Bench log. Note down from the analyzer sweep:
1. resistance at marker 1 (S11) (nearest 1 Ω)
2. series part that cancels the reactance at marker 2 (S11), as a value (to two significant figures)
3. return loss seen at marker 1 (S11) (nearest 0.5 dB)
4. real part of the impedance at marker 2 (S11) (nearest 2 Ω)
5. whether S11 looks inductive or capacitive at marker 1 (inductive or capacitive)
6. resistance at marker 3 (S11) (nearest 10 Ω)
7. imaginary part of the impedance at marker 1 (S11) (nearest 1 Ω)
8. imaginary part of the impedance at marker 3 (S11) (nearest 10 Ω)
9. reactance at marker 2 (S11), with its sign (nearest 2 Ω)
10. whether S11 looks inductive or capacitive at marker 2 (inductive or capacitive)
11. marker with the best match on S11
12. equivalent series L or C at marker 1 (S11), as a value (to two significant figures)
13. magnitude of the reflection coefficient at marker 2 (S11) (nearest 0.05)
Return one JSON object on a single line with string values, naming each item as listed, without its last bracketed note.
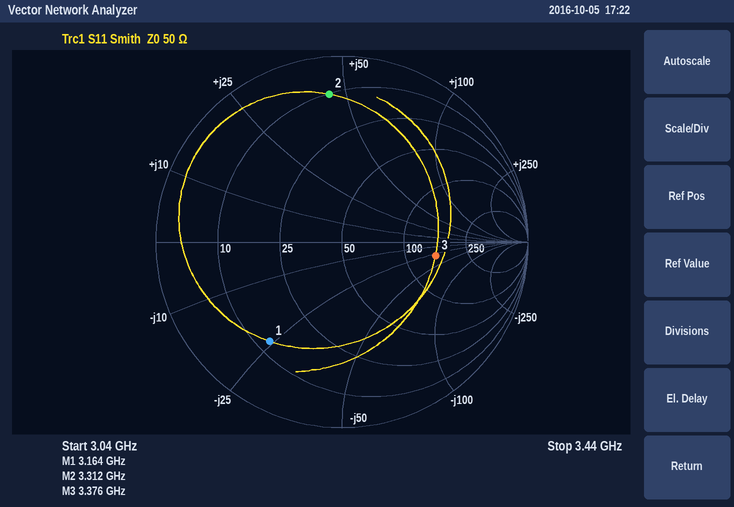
{"resistance at marker 1 (S11)": "13 Ω", "series part that cancels the reactance at marker 2 (S11), as a value": "1.1 pF", "return loss seen at marker 1 (S11)": "3.5 dB", "real part of the impedance at marker 2 (S11)": "10 Ω", "whether S11 looks inductive or capacitive at marker 1": "capacitive", "resistance at marker 3 (S11)": "150 Ω", "imaginary part of the impedance at marker 1 (S11)": "-24 Ω", "imaginary part of the impedance at marker 3 (S11)": "-30 Ω", "reactance at marker 2 (S11), with its sign": "+44 Ω", "whether S11 looks inductive or capacitive at marker 2": "inductive", "marker with the best match on S11": "marker 3", "equivalent series L or C at marker 1 (S11), as a value": "2.1 pF", "magnitude of the reflection coefficient at marker 2 (S11)": "0.80"}
